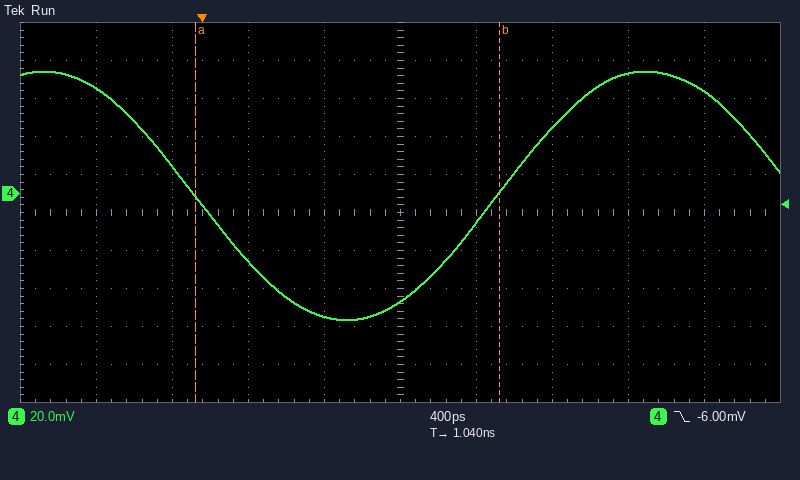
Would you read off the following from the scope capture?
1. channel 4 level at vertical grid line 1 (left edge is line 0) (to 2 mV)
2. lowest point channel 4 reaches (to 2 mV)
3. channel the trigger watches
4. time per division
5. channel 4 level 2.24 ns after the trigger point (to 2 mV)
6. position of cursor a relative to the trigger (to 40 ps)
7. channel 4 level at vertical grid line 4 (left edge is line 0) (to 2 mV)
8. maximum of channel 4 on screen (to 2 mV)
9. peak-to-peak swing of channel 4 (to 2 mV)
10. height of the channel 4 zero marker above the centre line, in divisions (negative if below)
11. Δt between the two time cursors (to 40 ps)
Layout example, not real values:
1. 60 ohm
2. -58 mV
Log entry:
1. 56 mV
2. -66 mV
3. channel 4
4. 400 ps
5. 64 mV
6. -40 ps
7. -64 mV
8. 64 mV
9. 130 mV
10. +0.5 div
11. 1.60 ns
